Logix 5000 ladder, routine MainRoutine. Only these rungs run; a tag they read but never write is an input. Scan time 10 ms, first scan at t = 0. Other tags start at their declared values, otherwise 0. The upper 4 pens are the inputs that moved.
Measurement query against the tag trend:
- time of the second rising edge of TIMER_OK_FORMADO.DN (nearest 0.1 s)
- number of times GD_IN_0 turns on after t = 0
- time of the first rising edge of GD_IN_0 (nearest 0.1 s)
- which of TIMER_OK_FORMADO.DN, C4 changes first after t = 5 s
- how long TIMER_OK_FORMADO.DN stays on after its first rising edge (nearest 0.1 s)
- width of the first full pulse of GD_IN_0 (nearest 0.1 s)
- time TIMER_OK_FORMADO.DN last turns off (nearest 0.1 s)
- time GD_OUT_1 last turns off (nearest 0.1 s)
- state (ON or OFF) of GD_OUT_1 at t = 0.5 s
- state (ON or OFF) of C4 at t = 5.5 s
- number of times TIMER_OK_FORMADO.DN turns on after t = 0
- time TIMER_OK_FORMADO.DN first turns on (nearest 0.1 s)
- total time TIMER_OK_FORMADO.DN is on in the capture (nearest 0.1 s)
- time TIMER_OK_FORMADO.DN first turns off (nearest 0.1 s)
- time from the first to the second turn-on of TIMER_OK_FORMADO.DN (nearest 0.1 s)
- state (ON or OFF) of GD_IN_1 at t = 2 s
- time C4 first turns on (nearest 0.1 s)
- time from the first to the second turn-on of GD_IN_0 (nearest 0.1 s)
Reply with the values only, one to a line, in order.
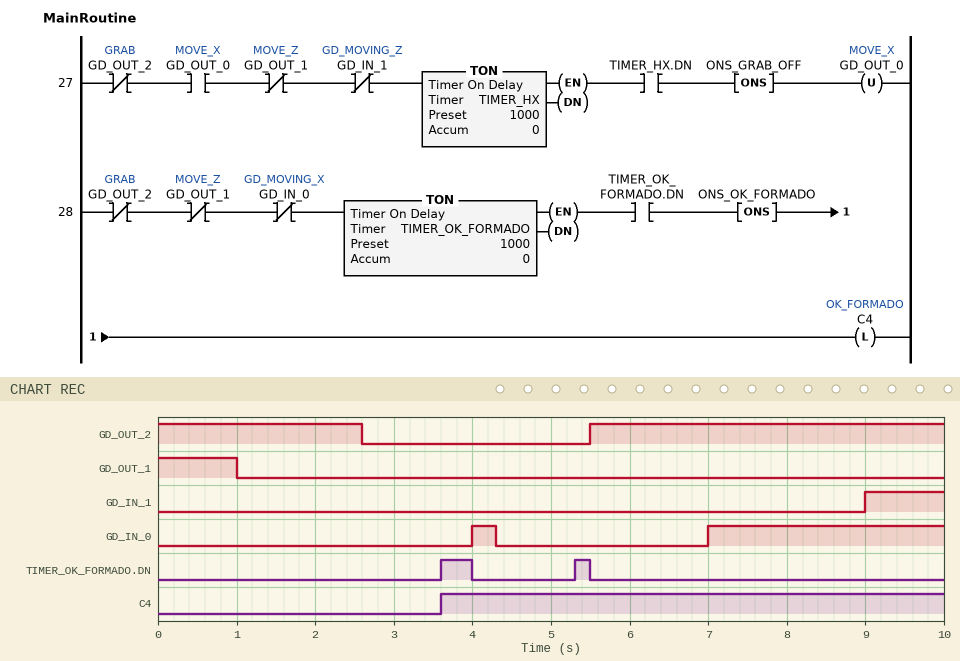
5.3 s
2
4.0 s
TIMER_OK_FORMADO.DN
0.4 s
0.3 s
5.5 s
1.0 s
ON
ON
2
3.6 s
0.6 s
4.0 s
1.7 s
OFF
3.6 s
3.0 s
